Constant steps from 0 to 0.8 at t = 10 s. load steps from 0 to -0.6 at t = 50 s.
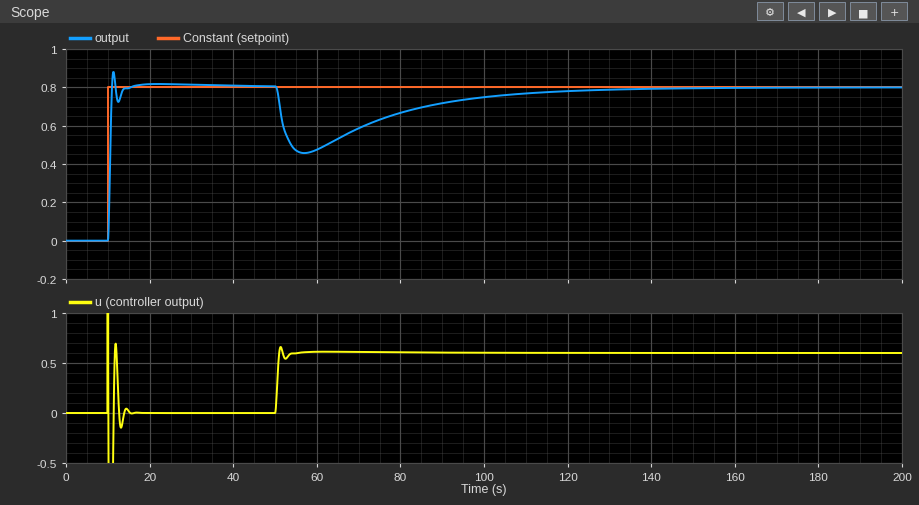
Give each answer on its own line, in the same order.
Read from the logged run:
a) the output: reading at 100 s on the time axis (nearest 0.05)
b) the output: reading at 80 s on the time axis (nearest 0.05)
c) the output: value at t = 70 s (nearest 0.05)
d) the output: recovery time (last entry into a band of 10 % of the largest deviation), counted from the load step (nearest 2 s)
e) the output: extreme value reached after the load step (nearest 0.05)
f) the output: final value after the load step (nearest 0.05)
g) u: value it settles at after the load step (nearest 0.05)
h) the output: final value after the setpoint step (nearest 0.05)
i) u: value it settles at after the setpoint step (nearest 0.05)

0.75
0.65
0.60
58 s
0.45
0.80
0.60
0.80
0.00
